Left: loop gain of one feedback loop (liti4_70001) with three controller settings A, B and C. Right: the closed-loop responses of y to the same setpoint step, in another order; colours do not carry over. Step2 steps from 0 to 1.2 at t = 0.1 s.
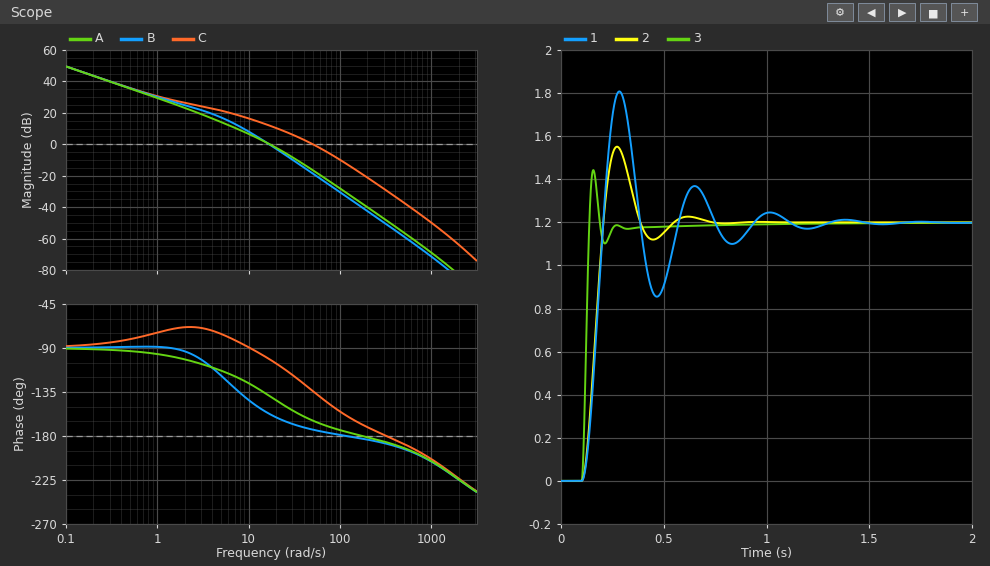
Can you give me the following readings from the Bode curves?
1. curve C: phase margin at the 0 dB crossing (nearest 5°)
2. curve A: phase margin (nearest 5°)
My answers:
45°
40°
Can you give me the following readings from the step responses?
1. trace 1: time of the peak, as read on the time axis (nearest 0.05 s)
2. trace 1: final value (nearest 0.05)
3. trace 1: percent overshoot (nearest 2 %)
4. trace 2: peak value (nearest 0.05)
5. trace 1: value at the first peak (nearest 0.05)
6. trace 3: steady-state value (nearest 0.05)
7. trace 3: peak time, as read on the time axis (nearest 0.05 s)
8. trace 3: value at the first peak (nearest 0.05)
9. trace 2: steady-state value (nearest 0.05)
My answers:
0.30 s
1.20
50 %
1.55
1.80
1.20
0.15 s
1.45
1.20
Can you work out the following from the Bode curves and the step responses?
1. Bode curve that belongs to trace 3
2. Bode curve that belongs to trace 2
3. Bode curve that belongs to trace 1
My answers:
C
A
B
